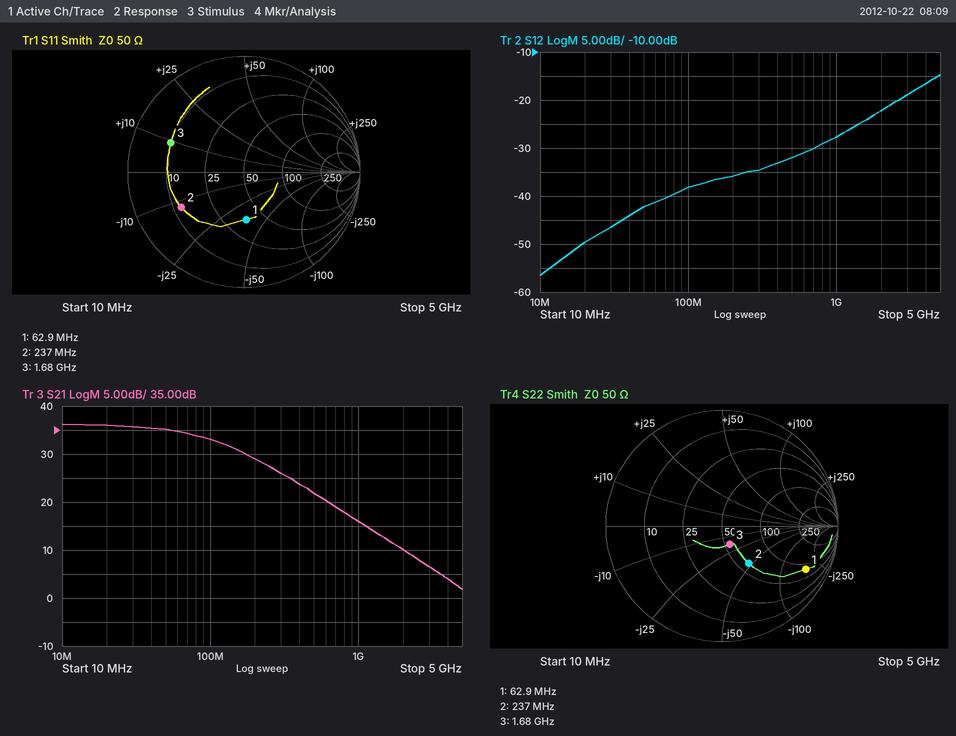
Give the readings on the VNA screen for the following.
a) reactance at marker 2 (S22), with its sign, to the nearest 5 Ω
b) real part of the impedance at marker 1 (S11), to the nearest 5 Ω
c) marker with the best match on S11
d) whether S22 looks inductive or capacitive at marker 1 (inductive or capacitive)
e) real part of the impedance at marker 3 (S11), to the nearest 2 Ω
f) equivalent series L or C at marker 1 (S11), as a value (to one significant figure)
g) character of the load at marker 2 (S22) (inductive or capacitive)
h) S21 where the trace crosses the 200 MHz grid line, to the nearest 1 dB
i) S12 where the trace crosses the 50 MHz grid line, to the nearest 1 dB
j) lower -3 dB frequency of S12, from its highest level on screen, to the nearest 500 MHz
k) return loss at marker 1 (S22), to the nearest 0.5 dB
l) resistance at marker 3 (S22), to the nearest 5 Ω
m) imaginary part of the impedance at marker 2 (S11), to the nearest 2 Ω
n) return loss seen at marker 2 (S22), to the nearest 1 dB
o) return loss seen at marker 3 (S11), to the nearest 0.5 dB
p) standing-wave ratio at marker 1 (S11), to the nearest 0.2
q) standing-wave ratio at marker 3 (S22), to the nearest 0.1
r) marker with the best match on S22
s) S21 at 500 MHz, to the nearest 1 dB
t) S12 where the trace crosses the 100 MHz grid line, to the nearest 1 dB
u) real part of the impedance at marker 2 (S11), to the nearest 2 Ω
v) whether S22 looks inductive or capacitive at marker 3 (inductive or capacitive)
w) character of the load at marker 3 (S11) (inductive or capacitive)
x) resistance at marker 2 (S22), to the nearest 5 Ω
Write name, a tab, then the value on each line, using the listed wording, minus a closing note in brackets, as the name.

reactance at marker 2 (S22), with its sign, to the nearest 5 Ω	-45 Ω
real part of the impedance at marker 1 (S11), to the nearest 5 Ω	35 Ω
marker with the best match on S11	marker 1
whether S22 looks inductive or capacitive at marker 1	capacitive
real part of the impedance at marker 3 (S11), to the nearest 2 Ω	10 Ω
equivalent series L or C at marker 1 (S11), as a value	70 pF
character of the load at marker 2 (S22)	capacitive
S21 where the trace crosses the 200 MHz grid line, to the nearest 1 dB	29 dB
S12 where the trace crosses the 50 MHz grid line, to the nearest 1 dB	-42 dB
lower -3 dB frequency of S12, from its highest level on screen, to the nearest 500 MHz	3.5 GHz
return loss at marker 1 (S22), to the nearest 0.5 dB	2.0 dB
resistance at marker 3 (S22), to the nearest 5 Ω	55 Ω
imaginary part of the impedance at marker 2 (S11), to the nearest 2 Ω	-12 Ω
return loss seen at marker 2 (S22), to the nearest 1 dB	8 dB
return loss seen at marker 3 (S11), to the nearest 0.5 dB	3.5 dB
standing-wave ratio at marker 1 (S11), to the nearest 0.2	2.4
standing-wave ratio at marker 3 (S22), to the nearest 0.1	1.4
marker with the best match on S22	marker 3
S21 at 500 MHz, to the nearest 1 dB	22 dB
S12 where the trace crosses the 100 MHz grid line, to the nearest 1 dB	-38 dB
real part of the impedance at marker 2 (S11), to the nearest 2 Ω	12 Ω
whether S22 looks inductive or capacitive at marker 3	capacitive
character of the load at marker 3 (S11)	inductive
resistance at marker 2 (S22), to the nearest 5 Ω	60 Ω
